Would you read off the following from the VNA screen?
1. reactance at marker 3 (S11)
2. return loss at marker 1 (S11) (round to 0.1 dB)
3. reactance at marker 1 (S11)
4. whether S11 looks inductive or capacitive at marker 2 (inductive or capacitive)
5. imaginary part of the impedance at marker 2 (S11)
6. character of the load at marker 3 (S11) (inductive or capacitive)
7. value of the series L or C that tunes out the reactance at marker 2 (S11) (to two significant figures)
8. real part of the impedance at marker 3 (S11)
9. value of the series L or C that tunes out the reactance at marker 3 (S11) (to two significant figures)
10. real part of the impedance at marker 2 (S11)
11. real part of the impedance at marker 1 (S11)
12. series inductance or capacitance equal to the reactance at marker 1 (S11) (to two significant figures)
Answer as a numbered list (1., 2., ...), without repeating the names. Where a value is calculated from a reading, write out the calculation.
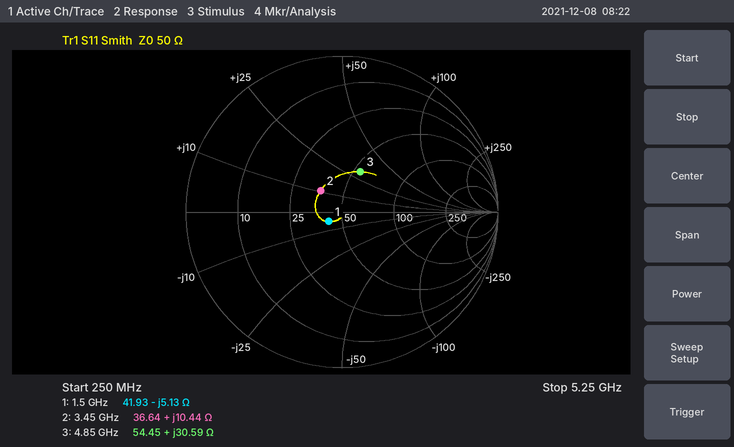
1. +30.59 Ω
2. 19.7 dB
3. -5.13 Ω
4. inductive
5. +10.44 Ω
6. inductive
7. C = 1/(2π × 3.45 GHz × 10.44 Ω) ≈ 4.4 pF
8. 54.45 Ω
9. C = 1/(2π × 4.85 GHz × 30.59 Ω) ≈ 1.1 pF
10. 36.64 Ω
11. 41.93 Ω
12. C = 1/(2π × 1.5 GHz × 5.13 Ω) ≈ 21 pF
